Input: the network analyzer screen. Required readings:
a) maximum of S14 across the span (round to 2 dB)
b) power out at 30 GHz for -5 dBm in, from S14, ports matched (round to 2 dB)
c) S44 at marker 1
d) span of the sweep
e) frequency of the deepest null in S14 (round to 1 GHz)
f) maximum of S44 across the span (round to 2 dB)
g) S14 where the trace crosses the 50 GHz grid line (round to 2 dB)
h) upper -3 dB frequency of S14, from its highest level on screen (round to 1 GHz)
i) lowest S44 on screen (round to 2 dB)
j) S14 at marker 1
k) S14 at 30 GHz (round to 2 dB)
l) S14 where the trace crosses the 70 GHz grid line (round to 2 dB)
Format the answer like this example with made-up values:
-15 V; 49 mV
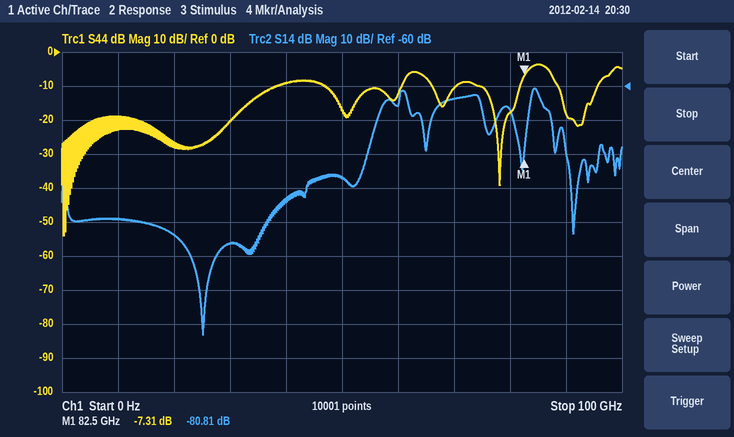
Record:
-60 dB; -112 dBm; -7.31 dB; 100 GHz; 25 GHz; -4 dB; -86 dB; 85 GHz; -54 dB; -80.81 dB; -106 dB; -64 dB
